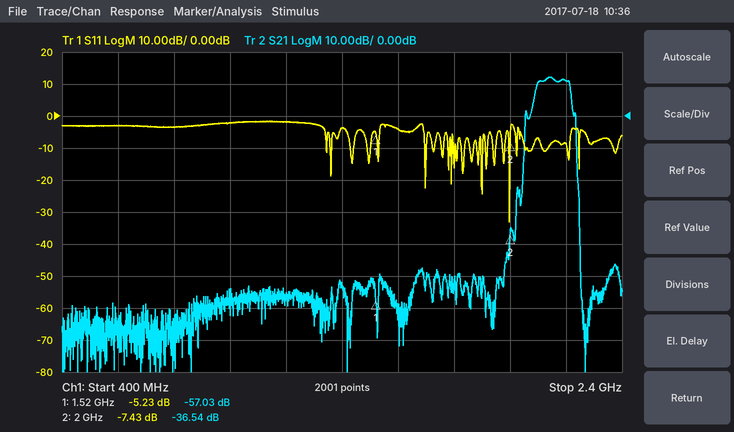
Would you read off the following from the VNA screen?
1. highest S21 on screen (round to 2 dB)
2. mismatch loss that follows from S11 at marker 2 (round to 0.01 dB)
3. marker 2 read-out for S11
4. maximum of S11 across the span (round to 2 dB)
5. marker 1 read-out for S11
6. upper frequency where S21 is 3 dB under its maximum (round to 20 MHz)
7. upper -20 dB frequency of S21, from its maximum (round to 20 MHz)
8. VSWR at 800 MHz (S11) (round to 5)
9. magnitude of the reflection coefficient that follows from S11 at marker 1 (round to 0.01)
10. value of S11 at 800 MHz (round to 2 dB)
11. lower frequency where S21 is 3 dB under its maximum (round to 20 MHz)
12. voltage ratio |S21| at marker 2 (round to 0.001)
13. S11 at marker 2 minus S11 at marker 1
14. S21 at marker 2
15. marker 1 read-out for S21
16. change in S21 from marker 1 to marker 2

12 dB
0.87 dB
-7.43 dB
-2 dB
-5.23 dB
2.22 GHz
2.24 GHz
5
0.55
-4 dB
2.10 GHz
0.015
-2.20 dB
-36.54 dB
-57.03 dB
20.49 dB
